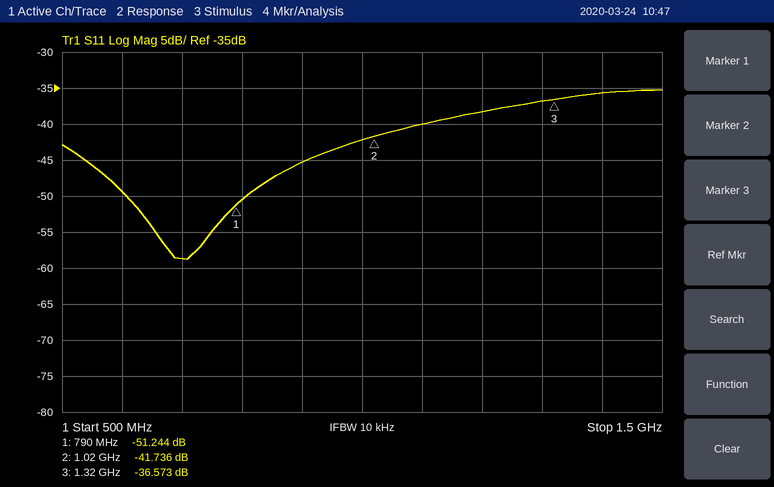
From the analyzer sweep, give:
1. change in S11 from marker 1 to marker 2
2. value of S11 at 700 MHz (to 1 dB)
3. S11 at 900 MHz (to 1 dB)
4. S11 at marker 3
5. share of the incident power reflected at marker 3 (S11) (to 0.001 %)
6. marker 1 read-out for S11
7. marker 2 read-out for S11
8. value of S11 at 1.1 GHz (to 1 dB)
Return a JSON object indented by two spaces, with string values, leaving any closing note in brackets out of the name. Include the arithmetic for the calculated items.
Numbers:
{
  "change in S11 from marker 1 to marker 2": "-41.736 − (-51.244) = 9.508 dB",
  "value of S11 at 700 MHz": "-59 dB",
  "S11 at 900 MHz": "-45 dB",
  "S11 at marker 3": "-36.573 dB",
  "share of the incident power reflected at marker 3 (S11)": "10^(-36.573/10) ≈ 0.022 %",
  "marker 1 read-out for S11": "-51.244 dB",
  "marker 2 read-out for S11": "-41.736 dB",
  "value of S11 at 1.1 GHz": "-40 dB"
}
